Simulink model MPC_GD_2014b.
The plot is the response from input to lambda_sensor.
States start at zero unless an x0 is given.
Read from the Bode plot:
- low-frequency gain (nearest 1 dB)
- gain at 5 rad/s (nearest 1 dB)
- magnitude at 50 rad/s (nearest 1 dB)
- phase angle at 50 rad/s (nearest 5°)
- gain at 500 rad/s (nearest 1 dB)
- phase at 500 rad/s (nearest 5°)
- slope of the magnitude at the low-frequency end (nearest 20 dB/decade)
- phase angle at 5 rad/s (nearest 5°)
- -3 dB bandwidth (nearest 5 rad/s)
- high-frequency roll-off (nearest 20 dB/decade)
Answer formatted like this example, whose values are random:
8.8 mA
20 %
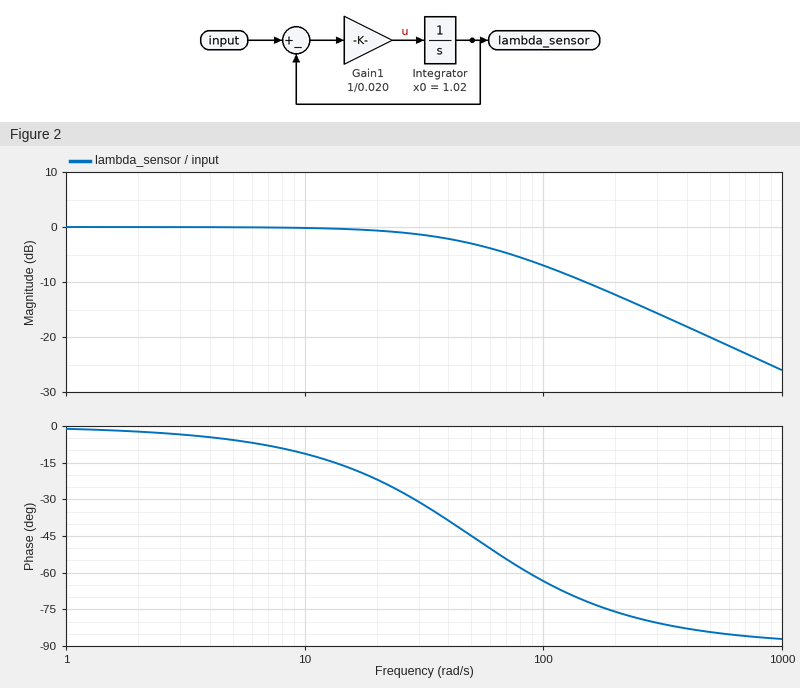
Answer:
0 dB
0 dB
-3 dB
-45°
-20 dB
-85°
0 dB/decade
-5°
50 rad/s
-20 dB/decade
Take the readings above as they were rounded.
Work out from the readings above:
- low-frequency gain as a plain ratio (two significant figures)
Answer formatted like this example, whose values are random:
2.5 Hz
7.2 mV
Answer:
1.0
